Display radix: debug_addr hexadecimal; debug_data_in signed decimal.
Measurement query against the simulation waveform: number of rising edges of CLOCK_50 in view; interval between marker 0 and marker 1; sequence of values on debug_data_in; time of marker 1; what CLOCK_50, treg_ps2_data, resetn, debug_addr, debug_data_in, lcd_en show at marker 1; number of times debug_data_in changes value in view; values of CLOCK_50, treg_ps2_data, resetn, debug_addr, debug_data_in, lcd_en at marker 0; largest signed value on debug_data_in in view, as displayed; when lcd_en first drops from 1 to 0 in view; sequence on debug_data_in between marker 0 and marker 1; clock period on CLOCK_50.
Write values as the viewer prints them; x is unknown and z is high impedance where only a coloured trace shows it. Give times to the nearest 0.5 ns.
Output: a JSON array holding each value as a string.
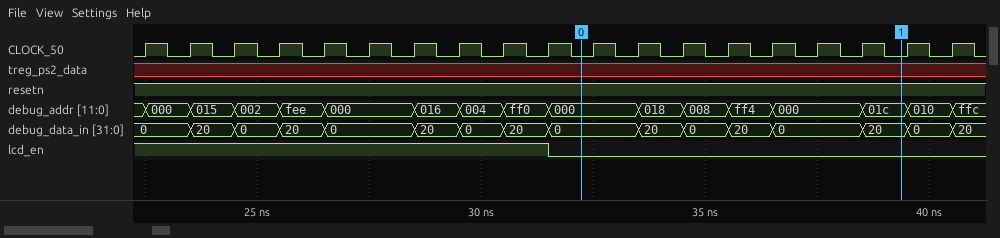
["19", "7 ns", "0, 20, 0, 20, 0, 20, 0, 20, 0, 20, 0, 20, 0, 20, 0, 20", "39.5 ns", "CLOCK_50=0, treg_ps2_data=x, resetn=1, debug_addr=01c, debug_data_in=20, lcd_en=0", "15", "CLOCK_50=0, treg_ps2_data=x, resetn=1, debug_addr=000, debug_data_in=0, lcd_en=0", "20", "31.5 ns", "0, 20, 0, 20, 0, 20", "1 ns"]
